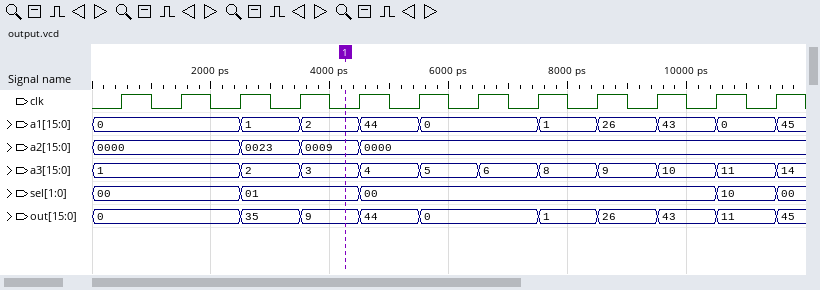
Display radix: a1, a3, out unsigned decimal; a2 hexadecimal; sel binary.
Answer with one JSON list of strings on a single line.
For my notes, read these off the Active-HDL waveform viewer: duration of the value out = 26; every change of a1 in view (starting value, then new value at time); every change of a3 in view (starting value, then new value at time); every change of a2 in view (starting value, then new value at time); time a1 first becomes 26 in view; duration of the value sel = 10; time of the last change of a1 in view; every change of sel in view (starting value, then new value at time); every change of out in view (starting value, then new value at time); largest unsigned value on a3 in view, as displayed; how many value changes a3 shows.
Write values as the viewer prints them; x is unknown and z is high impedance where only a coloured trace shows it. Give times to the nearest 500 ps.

["1000 ps", "0, 1 at 2500 ps, 2 at 3500 ps, 44 at 4500 ps, 0 at 5500 ps, 1 at 7500 ps, 26 at 8500 ps, 43 at 9500 ps, 0 at 10500 ps, 45 at 11500 ps", "1, 2 at 2500 ps, 3 at 3500 ps, 4 at 4500 ps, 5 at 5500 ps, 6 at 6500 ps, 8 at 7500 ps, 9 at 8500 ps, 10 at 9500 ps, 11 at 10500 ps, 14 at 11500 ps", "0000, 0023 at 2500 ps, 0009 at 3500 ps, 0000 at 4500 ps", "8500 ps", "1000 ps", "11500 ps", "00, 01 at 2500 ps, 00 at 4500 ps, 10 at 10500 ps, 00 at 11500 ps", "0, 35 at 2500 ps, 9 at 3500 ps, 44 at 4500 ps, 0 at 5500 ps, 1 at 7500 ps, 26 at 8500 ps, 43 at 9500 ps, 11 at 10500 ps, 45 at 11500 ps", "14", "10"]
